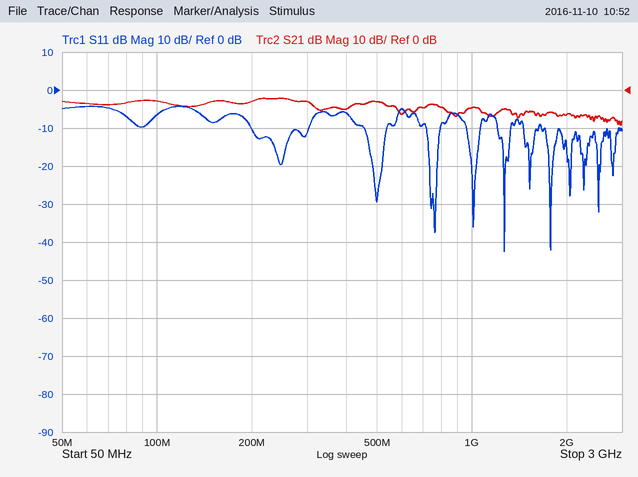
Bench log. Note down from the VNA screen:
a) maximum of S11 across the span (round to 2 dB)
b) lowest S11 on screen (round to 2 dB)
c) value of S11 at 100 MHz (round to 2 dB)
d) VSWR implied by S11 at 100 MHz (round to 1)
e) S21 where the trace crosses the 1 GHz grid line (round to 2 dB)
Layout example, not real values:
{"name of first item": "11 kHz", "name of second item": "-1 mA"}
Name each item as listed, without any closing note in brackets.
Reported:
{"maximum of S11 across the span": "-4 dB", "lowest S11 on screen": "-42 dB", "value of S11 at 100 MHz": "-6 dB", "VSWR implied by S11 at 100 MHz": "3", "S21 where the trace crosses the 1 GHz grid line": "-4 dB"}
